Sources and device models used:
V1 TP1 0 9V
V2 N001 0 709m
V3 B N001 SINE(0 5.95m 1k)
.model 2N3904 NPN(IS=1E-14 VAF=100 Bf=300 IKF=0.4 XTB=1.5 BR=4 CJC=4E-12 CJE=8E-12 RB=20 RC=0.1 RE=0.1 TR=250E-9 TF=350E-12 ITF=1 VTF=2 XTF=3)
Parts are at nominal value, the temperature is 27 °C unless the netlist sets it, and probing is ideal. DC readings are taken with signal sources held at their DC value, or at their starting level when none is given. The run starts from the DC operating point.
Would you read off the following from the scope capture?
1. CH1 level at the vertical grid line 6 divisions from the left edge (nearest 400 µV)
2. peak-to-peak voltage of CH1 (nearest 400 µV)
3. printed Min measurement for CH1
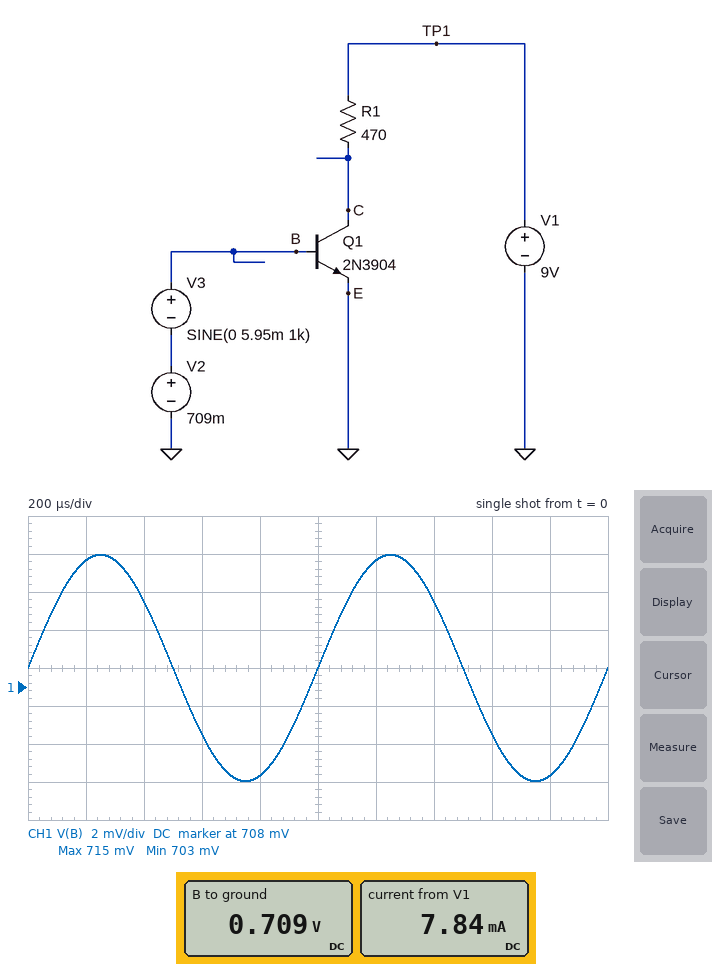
714.8 mV
12.0 mV
703 mV
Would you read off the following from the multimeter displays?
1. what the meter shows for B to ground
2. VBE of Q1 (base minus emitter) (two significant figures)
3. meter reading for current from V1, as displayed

0.709 V
710 mV
7.84 mA
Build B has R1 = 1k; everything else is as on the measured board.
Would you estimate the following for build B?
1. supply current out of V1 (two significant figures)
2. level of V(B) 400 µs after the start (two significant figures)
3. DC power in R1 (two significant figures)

7.6 mA
710 mV
57 mW
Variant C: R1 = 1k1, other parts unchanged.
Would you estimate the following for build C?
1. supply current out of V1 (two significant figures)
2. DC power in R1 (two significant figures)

7.5 mA
62 mW
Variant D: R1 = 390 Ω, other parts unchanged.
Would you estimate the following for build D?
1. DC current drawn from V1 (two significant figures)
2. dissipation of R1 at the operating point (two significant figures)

7.9 mA
24 mW
